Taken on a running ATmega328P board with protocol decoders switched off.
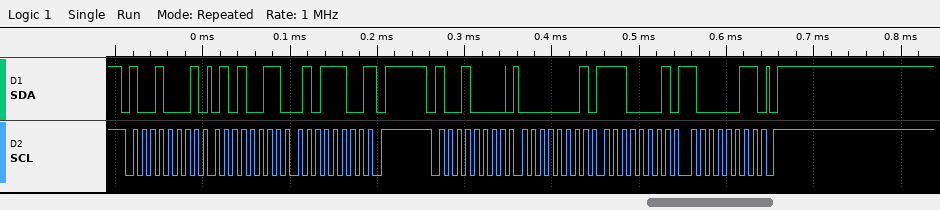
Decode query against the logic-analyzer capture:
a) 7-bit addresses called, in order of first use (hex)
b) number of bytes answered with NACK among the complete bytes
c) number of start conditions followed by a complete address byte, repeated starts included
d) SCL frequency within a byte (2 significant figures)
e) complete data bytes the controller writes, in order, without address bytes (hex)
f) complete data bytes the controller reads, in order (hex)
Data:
0x48
1
2
100 kHz
01 E1 83
53 5C
